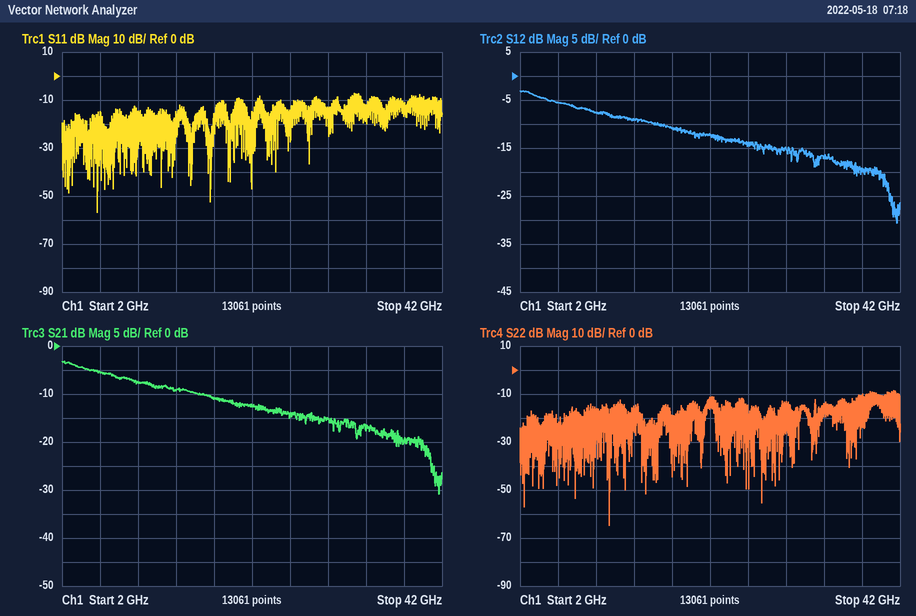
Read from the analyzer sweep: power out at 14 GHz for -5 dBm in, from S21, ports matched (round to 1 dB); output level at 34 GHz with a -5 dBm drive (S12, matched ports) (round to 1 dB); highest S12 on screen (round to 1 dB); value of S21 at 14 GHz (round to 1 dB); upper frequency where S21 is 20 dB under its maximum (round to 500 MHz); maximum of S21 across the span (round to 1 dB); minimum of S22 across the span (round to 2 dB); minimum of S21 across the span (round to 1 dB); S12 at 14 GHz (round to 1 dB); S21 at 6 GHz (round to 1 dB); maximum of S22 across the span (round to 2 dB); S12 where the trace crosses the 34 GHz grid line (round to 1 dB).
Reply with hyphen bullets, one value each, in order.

- -14 dBm
- -22 dBm
- -3 dB
- -9 dB
- 40.5 GHz
- -3 dB
- -64 dB
- -31 dB
- -9 dB
- -5 dB
- -8 dB
- -17 dB
